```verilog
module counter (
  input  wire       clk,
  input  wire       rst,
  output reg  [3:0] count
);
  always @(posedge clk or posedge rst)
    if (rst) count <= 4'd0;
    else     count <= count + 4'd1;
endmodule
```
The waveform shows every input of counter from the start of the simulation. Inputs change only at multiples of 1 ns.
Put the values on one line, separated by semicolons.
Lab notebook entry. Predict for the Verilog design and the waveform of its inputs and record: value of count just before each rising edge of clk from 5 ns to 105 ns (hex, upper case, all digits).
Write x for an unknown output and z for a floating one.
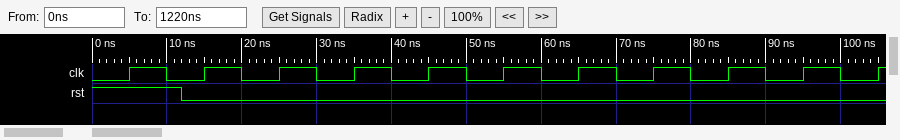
0, 0, 1, 2, 3, 4, 5, 6, 7, 8, 9
